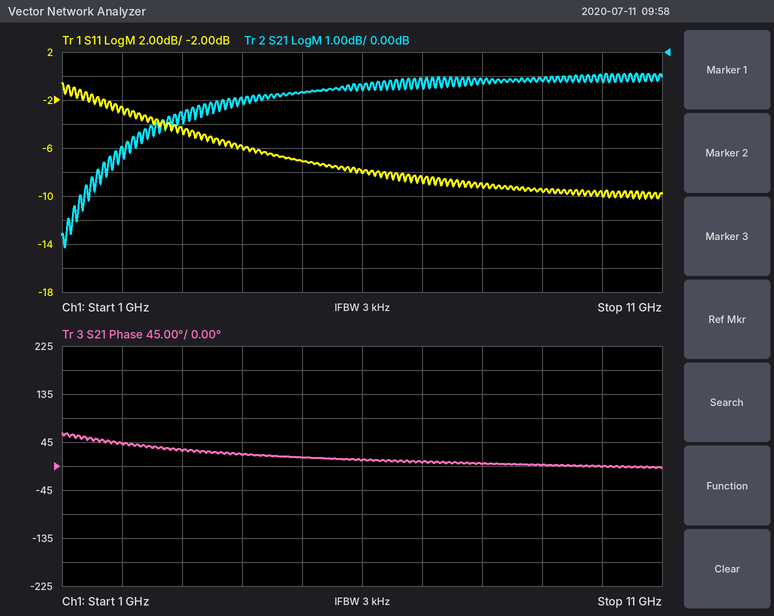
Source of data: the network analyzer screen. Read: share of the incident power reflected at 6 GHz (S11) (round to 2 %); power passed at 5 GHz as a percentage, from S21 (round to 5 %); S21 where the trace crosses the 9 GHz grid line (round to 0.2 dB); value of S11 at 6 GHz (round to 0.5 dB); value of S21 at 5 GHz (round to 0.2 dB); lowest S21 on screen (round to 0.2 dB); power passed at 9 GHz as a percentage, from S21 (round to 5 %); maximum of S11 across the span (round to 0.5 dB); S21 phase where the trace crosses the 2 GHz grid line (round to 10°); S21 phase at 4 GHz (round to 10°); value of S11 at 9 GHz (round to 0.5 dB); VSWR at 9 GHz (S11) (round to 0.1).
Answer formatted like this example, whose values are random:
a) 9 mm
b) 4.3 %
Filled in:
a) 16 %
b) 70 %
c) -1.2 dB
d) -8.0 dB
e) -1.6 dB
f) -8.2 dB
g) 75 %
h) -0.5 dB
i) 40°
j) 20°
k) -9.5 dB
l) 2.0
